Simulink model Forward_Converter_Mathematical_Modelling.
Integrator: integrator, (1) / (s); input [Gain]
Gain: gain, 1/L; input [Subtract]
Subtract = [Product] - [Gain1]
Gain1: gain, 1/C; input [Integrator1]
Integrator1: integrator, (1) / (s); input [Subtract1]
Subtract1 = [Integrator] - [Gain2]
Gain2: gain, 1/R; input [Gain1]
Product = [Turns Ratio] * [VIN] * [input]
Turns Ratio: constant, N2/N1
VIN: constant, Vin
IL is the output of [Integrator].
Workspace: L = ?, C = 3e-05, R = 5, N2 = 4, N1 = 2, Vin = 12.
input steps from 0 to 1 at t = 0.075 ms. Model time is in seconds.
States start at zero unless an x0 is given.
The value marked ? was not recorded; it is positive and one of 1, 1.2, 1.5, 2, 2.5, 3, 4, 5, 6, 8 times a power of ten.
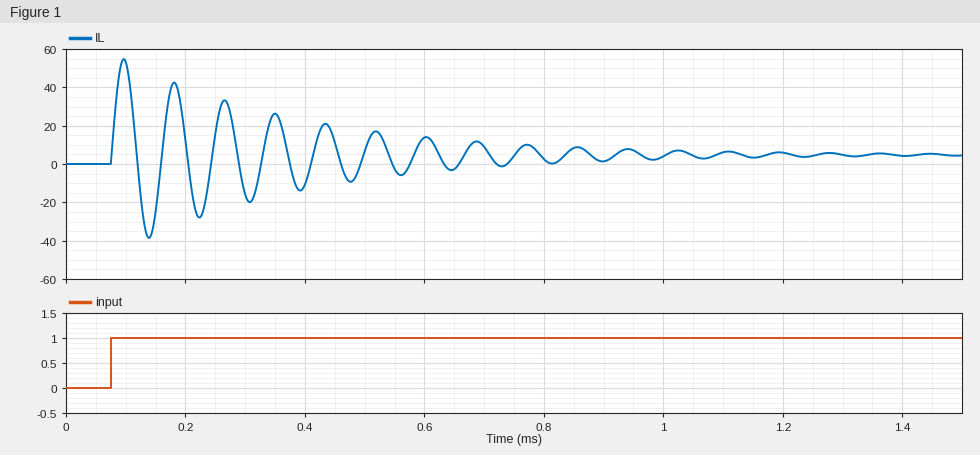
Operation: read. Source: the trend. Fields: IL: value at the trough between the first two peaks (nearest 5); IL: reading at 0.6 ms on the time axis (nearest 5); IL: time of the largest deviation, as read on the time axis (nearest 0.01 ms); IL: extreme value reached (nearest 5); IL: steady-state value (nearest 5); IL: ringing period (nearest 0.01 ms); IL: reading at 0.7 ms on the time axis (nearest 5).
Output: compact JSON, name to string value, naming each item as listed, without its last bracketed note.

{"IL: value at the trough between the first two peaks": "-40", "IL: reading at 0.6 ms on the time axis": "15", "IL: time of the largest deviation, as read on the time axis": "0.10 ms", "IL: extreme value reached": "55", "IL: steady-state value": "5", "IL: ringing period": "0.08 ms", "IL: reading at 0.7 ms on the time axis": "10"}
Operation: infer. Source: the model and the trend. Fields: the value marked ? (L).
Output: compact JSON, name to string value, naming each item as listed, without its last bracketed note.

{"the value marked ?": "6e-06"}
